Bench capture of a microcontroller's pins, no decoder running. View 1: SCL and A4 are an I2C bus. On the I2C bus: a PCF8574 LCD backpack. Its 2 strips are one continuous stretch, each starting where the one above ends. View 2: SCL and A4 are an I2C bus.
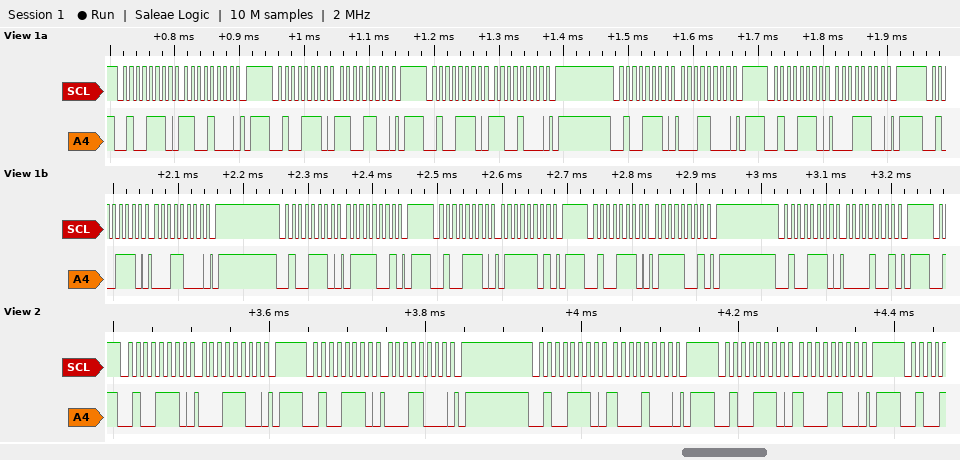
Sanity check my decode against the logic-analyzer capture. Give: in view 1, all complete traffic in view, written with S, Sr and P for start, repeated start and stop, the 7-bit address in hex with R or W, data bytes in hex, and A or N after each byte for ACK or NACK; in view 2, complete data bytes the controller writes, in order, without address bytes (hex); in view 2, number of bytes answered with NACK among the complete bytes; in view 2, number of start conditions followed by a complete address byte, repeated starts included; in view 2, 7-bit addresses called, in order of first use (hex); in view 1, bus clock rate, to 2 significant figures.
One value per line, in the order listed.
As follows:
S 27W A C8 A P S 27W A CC A P S 27W A C8 A P S 27W A 18 A P S 27W A 1C A P S 27W A 18 A P S 27W A 79 A P S 27W A 7D A P S 27W A 79 A P S 27W A 09 A P
1C 18 88 8C
0
4
0x27
100 kHz
